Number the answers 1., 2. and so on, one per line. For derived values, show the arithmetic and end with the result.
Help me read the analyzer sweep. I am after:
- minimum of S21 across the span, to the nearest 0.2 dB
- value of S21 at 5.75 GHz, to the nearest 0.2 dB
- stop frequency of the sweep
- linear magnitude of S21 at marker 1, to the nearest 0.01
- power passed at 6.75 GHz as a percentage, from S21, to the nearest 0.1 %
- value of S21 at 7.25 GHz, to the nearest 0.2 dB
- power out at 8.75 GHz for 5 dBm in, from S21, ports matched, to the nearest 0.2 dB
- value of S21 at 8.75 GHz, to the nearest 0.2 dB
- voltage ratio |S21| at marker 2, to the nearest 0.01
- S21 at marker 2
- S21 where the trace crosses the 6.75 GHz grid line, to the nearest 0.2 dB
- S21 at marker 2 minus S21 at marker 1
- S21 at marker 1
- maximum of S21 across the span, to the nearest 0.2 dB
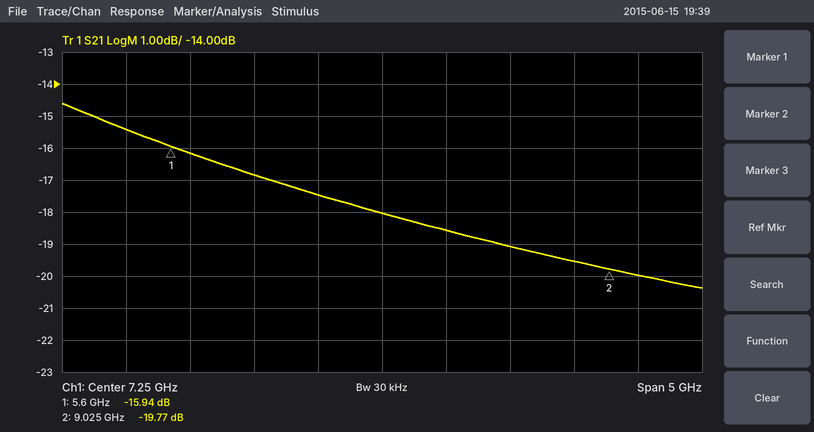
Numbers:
1. -20.4 dB
2. -16.2 dB
3. 9.75 GHz
4. 10^(-15.94/20) ≈ 0.16
5. 10^(-17.4/10) ≈ 1.8 %
6. -18.0 dB
7. 5 dBm + (-19.6 dB) = -14.6 dBm
8. -19.6 dB
9. 10^(-19.77/20) ≈ 0.10
10. -19.77 dB
11. -17.4 dB
12. -19.77 − (-15.94) = -3.83 dB
13. -15.94 dB
14. -14.6 dB
